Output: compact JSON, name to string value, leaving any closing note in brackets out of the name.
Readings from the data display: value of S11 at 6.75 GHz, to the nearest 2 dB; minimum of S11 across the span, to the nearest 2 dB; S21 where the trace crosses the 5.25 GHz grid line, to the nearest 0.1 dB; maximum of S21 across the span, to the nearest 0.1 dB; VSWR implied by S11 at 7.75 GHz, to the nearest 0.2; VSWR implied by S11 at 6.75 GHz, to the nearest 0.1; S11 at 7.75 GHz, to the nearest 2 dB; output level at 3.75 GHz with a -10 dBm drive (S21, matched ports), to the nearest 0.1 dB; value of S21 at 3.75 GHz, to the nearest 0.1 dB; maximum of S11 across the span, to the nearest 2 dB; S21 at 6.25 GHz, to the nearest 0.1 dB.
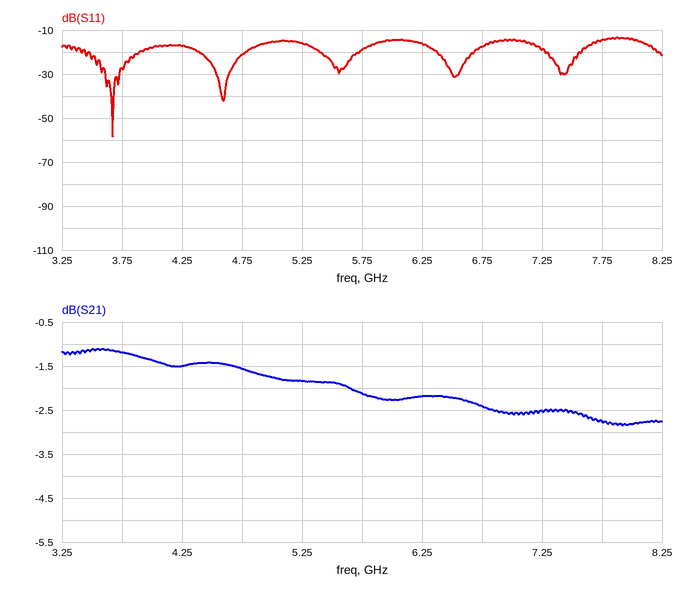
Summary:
{"value of S11 at 6.75 GHz, to the nearest 2 dB": "-18 dB", "minimum of S11 across the span, to the nearest 2 dB": "-58 dB", "S21 where the trace crosses the 5.25 GHz grid line, to the nearest 0.1 dB": "-1.8 dB", "maximum of S21 across the span, to the nearest 0.1 dB": "-1.1 dB", "VSWR implied by S11 at 7.75 GHz, to the nearest 0.2": "1.4", "VSWR implied by S11 at 6.75 GHz, to the nearest 0.1": "1.3", "S11 at 7.75 GHz, to the nearest 2 dB": "-14 dB", "output level at 3.75 GHz with a -10 dBm drive (S21, matched ports), to the nearest 0.1 dB": "-11.2 dBm", "value of S21 at 3.75 GHz, to the nearest 0.1 dB": "-1.2 dB", "maximum of S11 across the span, to the nearest 2 dB": "-14 dB", "S21 at 6.25 GHz, to the nearest 0.1 dB": "-2.2 dB"}
